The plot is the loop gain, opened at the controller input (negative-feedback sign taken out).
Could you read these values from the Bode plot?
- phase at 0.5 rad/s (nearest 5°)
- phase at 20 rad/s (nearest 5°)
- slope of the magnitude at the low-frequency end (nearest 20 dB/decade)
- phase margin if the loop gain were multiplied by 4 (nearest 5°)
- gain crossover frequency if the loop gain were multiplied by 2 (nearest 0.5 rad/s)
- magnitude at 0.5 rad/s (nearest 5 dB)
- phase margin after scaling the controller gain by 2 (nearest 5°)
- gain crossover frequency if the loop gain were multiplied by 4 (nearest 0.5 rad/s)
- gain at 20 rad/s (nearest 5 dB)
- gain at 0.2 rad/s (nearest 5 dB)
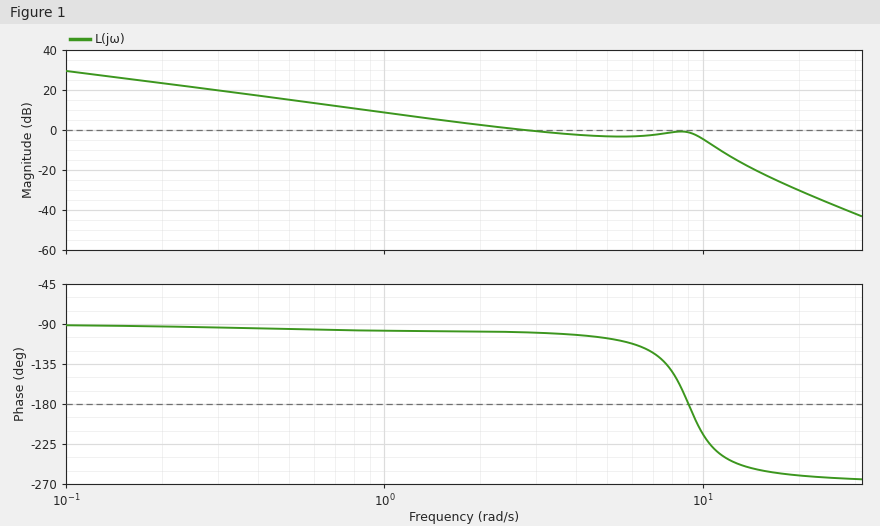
-95°
-260°
-20 dB/decade
-60°
10.5 rad/s
15 dB
-40°
12.0 rad/s
-30 dB
25 dB
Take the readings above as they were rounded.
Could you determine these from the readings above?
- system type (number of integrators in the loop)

1
